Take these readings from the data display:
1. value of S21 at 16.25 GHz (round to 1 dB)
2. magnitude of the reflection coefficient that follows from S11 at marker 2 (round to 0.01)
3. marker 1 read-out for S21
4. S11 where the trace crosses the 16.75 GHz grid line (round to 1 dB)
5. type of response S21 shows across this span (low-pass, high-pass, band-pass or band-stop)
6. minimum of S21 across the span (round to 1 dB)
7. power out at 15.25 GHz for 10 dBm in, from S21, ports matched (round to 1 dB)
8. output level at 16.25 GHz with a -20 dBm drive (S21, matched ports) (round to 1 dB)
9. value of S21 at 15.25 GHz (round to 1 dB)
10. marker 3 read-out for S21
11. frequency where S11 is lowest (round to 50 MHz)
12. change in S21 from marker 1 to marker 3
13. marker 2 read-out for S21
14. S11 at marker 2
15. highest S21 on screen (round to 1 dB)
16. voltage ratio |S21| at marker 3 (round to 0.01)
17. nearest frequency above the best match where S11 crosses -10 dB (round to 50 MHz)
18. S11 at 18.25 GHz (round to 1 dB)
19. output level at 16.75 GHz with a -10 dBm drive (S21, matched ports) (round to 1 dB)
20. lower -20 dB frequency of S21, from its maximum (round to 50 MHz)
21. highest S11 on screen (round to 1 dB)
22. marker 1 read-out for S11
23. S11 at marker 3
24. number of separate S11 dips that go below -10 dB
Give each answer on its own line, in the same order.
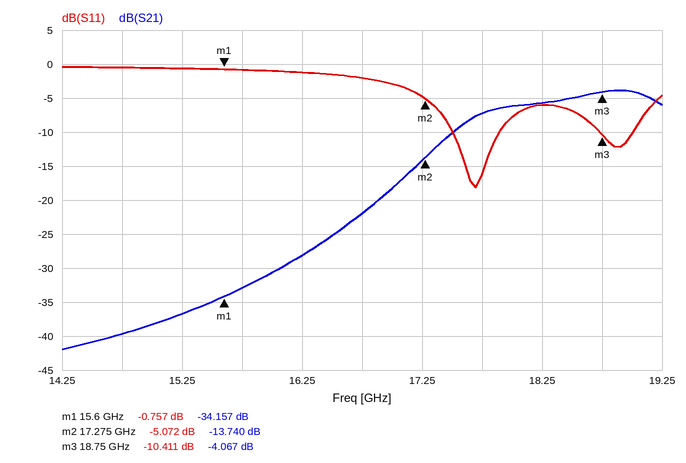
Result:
-28 dB
0.56
-34.157 dB
-2 dB
high-pass
-42 dB
-27 dBm
-48 dBm
-37 dB
-4.067 dB
17.70 GHz
30.090 dB
-13.740 dB
-5.072 dB
-4 dB
0.63
17.90 GHz
-6 dB
-32 dBm
16.60 GHz
0 dB
-0.757 dB
-10.411 dB
2
